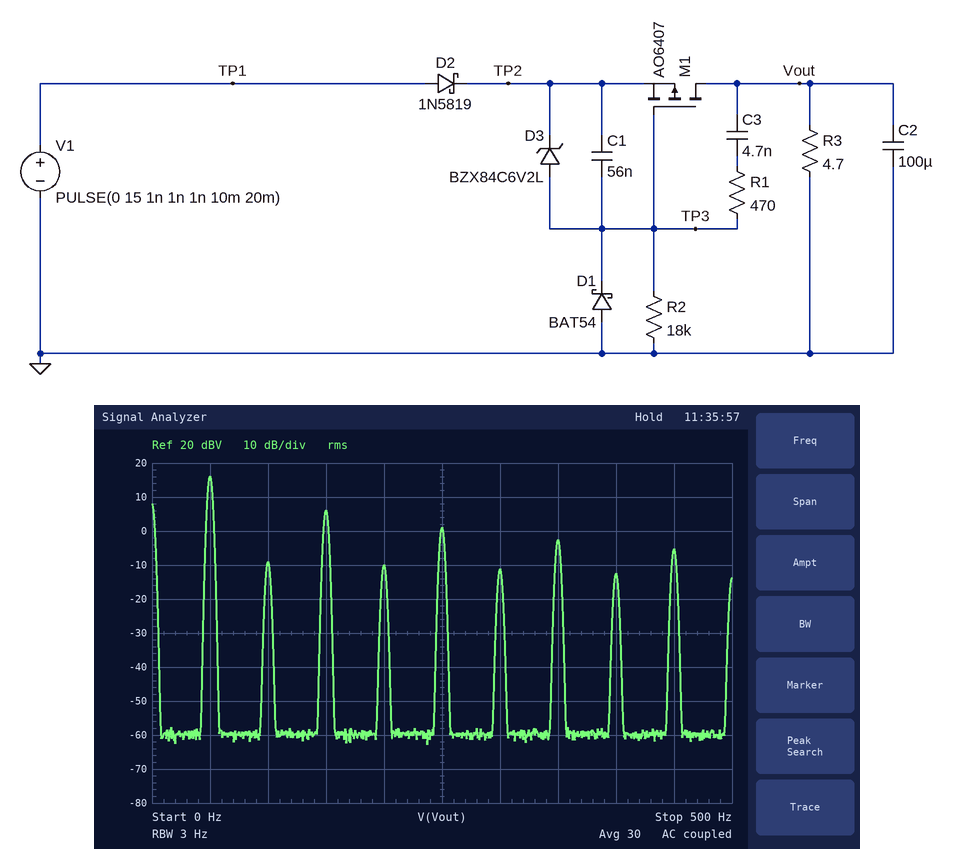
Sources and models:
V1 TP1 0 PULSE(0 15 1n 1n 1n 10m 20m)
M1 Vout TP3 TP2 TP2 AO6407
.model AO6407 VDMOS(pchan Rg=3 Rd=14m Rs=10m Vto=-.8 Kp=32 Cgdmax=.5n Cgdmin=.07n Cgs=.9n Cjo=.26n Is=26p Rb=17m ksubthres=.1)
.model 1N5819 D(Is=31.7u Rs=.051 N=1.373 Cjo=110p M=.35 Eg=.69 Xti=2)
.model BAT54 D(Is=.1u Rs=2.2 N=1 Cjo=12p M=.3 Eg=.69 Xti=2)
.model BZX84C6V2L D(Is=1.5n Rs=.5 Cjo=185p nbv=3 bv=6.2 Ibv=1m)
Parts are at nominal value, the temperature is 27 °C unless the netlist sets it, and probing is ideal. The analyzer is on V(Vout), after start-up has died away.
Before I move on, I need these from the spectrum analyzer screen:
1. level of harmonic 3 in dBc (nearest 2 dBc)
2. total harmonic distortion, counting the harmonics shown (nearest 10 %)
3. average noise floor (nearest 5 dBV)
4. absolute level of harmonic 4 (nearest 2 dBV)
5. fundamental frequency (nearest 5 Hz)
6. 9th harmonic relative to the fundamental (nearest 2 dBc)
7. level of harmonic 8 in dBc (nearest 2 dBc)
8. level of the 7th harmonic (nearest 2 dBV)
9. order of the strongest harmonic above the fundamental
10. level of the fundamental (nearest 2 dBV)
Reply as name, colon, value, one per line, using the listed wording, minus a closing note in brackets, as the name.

level of harmonic 3 in dBc: -10 dBc
total harmonic distortion, counting the harmonics shown: 40 %
average noise floor: -60 dBV
absolute level of harmonic 4: -10 dBV
fundamental frequency: 50 Hz
9th harmonic relative to the fundamental: -22 dBc
level of harmonic 8 in dBc: -28 dBc
level of the 7th harmonic: -2 dBV
order of the strongest harmonic above the fundamental: 3
level of the fundamental: 16 dBV
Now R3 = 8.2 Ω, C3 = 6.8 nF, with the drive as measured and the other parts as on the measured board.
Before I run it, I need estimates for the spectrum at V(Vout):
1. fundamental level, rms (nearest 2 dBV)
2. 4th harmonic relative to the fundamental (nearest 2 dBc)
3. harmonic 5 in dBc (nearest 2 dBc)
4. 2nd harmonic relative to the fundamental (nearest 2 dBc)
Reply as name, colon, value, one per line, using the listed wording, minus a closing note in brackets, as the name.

fundamental level, rms: 16 dBV
4th harmonic relative to the fundamental: -22 dBc
harmonic 5 in dBc: -16 dBc
2nd harmonic relative to the fundamental: -20 dBc
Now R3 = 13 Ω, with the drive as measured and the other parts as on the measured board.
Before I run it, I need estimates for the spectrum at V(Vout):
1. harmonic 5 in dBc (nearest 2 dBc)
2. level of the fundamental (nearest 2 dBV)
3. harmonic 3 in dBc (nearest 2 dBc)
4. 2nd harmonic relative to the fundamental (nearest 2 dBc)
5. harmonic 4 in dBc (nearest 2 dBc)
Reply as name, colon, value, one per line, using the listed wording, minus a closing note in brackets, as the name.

harmonic 5 in dBc: -18 dBc
level of the fundamental: 16 dBV
harmonic 3 in dBc: -12 dBc
2nd harmonic relative to the fundamental: -16 dBc
harmonic 4 in dBc: -20 dBc
